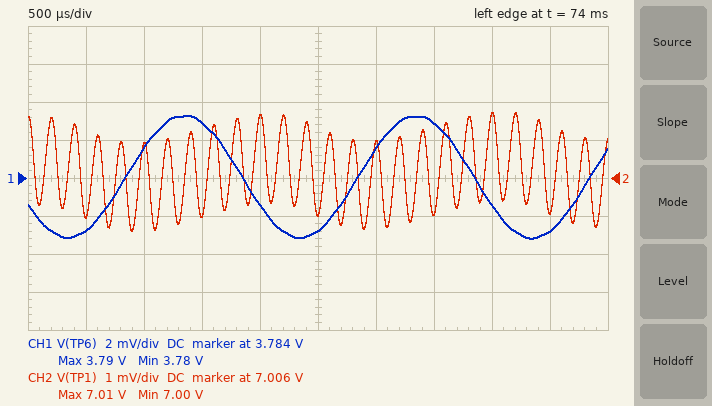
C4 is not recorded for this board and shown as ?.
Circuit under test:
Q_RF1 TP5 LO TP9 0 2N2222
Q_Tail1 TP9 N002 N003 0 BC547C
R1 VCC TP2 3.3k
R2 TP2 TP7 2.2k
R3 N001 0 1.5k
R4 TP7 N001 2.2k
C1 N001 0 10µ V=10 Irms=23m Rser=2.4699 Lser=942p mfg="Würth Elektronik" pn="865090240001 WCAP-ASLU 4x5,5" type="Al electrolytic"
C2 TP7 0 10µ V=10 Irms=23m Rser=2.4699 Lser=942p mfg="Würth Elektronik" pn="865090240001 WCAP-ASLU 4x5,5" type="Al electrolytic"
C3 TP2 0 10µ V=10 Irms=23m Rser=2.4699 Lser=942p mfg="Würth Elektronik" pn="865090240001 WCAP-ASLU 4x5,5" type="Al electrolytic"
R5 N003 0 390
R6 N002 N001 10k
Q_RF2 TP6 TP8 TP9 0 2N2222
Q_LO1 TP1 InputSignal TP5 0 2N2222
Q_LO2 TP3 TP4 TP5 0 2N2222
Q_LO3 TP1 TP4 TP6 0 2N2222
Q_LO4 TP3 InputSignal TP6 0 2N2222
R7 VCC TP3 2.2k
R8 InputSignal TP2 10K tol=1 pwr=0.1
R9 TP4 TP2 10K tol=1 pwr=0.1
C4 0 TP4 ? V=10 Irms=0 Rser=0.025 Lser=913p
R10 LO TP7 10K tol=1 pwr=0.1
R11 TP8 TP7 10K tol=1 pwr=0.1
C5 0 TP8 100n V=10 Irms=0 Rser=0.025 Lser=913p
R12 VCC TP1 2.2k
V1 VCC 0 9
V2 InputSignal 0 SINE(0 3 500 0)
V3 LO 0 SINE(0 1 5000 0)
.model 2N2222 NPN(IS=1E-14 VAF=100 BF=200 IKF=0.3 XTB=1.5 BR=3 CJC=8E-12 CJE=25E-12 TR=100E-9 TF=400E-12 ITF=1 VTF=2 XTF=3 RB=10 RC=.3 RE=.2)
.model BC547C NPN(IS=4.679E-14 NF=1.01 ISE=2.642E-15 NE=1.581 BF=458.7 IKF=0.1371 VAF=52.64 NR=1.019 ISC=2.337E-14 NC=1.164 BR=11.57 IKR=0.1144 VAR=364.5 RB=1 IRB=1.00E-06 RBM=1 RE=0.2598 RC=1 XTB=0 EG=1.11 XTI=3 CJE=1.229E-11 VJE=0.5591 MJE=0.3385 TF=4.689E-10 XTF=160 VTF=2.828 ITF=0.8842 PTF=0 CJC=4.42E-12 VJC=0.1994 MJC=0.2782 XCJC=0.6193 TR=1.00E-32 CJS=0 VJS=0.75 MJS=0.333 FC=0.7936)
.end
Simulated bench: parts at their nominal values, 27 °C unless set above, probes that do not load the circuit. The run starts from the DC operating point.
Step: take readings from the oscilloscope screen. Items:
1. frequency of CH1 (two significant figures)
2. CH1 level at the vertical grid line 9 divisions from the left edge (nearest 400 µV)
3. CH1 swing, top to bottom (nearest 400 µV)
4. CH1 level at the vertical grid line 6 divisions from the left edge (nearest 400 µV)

500 Hz
3.7812 V
6.4 mV
3.7856 V
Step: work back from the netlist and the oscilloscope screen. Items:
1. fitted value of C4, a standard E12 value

82 nF
